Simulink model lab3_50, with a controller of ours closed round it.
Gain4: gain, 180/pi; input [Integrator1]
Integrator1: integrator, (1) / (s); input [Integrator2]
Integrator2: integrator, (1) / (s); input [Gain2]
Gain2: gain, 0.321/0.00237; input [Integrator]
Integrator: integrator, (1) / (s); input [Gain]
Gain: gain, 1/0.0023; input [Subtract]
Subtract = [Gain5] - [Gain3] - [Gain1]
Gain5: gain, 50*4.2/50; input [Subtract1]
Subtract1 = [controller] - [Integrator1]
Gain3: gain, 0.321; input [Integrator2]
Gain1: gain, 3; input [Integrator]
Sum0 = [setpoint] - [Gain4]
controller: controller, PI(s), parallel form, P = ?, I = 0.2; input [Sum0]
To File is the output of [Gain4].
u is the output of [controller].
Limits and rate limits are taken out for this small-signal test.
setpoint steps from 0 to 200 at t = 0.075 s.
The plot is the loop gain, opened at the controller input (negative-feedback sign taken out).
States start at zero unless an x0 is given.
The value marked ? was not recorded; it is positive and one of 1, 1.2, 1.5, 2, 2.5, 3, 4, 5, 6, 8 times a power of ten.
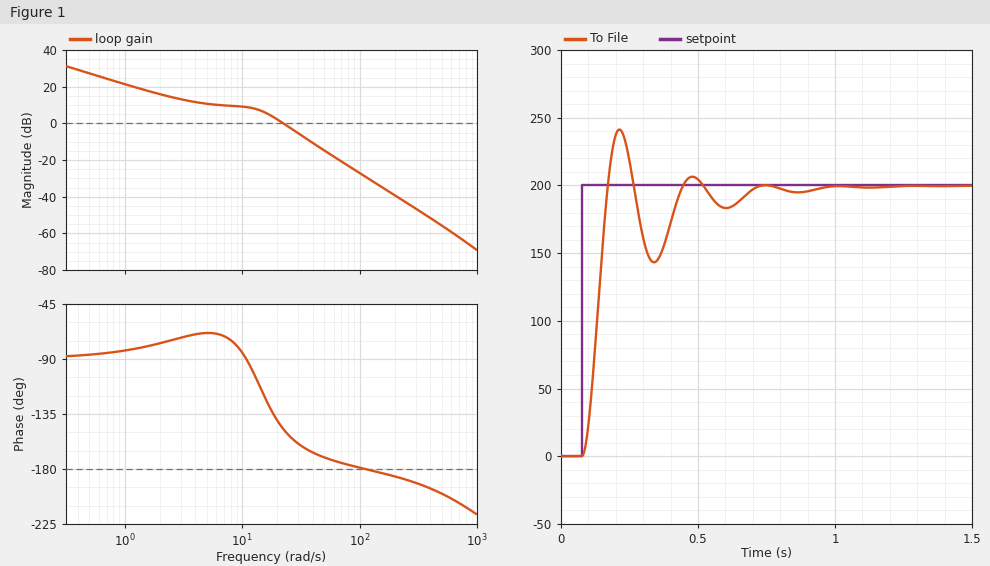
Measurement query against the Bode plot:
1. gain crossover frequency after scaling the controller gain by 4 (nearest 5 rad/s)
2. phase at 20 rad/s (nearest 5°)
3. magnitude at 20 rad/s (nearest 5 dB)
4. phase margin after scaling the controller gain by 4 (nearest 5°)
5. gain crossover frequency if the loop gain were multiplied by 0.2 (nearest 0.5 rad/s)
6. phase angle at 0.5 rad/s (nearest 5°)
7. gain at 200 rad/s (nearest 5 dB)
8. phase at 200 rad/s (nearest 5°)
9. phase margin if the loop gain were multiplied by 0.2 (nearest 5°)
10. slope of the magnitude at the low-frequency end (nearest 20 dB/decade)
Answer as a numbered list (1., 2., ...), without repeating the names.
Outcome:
1. 45 rad/s
2. -140°
3. 0 dB
4. 10°
5. 2.5 rad/s
6. -85°
7. -40 dB
8. -185°
9. 105°
10. -20 dB/decade
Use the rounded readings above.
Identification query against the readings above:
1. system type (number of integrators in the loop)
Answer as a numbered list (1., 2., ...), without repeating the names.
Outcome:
1. 1
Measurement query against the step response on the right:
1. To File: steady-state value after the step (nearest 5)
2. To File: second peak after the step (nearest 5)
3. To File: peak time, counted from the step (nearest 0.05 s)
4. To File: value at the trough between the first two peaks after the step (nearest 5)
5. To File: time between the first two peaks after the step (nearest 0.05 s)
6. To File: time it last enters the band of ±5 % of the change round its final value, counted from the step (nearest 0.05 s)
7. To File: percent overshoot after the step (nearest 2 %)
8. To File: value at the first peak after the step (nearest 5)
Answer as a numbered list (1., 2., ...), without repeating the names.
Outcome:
1. 200
2. 205
3. 0.15 s
4. 145
5. 0.25 s
6. 0.60 s
7. 20 %
8. 240
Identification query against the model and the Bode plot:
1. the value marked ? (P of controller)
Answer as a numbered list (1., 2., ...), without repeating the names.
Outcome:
1. 0.04
